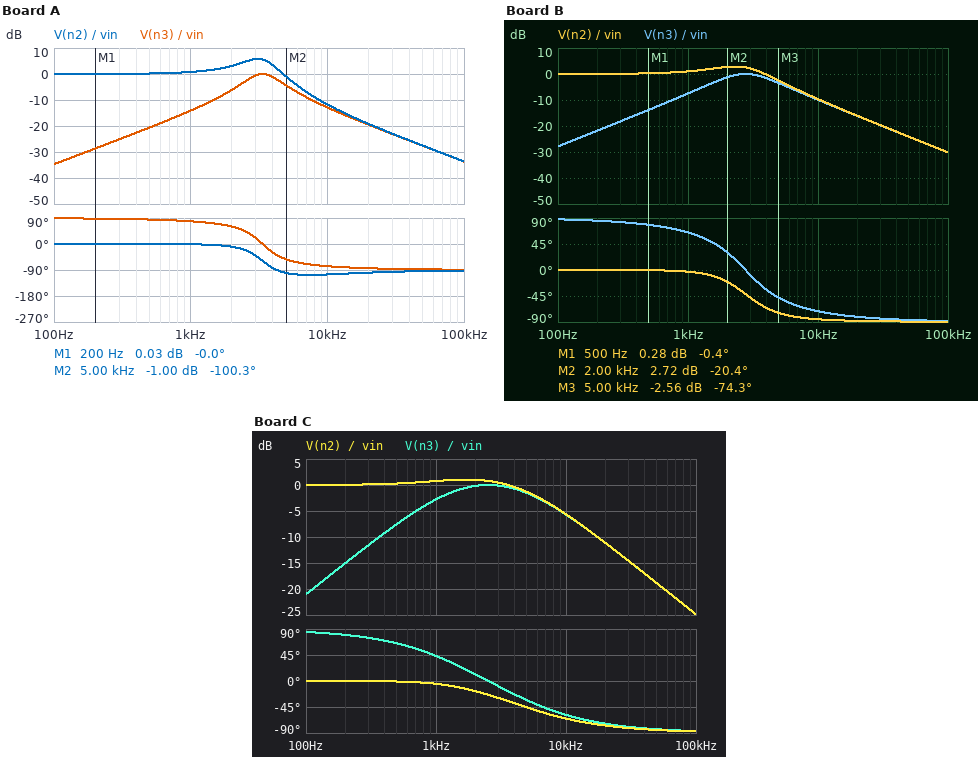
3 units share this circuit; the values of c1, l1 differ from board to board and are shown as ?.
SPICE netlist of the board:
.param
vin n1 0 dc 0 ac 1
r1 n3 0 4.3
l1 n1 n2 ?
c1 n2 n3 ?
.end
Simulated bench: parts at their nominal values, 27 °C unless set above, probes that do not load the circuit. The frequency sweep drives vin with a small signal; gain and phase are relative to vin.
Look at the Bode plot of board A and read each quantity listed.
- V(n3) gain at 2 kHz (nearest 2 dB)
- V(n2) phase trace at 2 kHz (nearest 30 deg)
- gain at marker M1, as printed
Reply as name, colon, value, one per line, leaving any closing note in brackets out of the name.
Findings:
V(n3) gain at 2 kHz: -6 dB
V(n2) phase trace at 2 kHz: 0 deg
gain at marker M1, as printed: 0.03 dB
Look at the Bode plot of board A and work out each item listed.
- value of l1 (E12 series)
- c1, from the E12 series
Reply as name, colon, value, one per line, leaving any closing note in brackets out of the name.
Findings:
value of l1: 330 µH
c1, from the E12 series: 6.8 µF
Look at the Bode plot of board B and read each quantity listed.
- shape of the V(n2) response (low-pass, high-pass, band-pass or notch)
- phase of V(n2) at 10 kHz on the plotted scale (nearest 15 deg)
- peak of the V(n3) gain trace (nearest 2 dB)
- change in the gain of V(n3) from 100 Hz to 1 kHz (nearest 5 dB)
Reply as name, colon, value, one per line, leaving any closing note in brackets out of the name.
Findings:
shape of the V(n2) response: low-pass
phase of V(n2) at 10 kHz on the plotted scale: -90 deg
peak of the V(n3) gain trace: 0 dB
change in the gain of V(n3) from 100 Hz to 1 kHz: 20 dB
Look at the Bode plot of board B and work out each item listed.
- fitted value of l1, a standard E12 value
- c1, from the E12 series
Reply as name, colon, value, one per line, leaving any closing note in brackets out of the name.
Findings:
fitted value of l1, a standard E12 value: 220 µH
c1, from the E12 series: 15 µF
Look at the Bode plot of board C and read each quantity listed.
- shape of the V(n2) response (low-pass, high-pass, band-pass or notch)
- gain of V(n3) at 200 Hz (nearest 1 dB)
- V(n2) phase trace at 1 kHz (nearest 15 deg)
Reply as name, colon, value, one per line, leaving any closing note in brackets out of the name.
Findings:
shape of the V(n2) response: low-pass
gain of V(n3) at 200 Hz: -15 dB
V(n2) phase trace at 1 kHz: 0 deg
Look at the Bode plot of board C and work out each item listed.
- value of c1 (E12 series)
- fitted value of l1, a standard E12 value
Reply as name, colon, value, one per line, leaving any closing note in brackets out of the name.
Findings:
value of c1: 33 µF
fitted value of l1, a standard E12 value: 120 µH
